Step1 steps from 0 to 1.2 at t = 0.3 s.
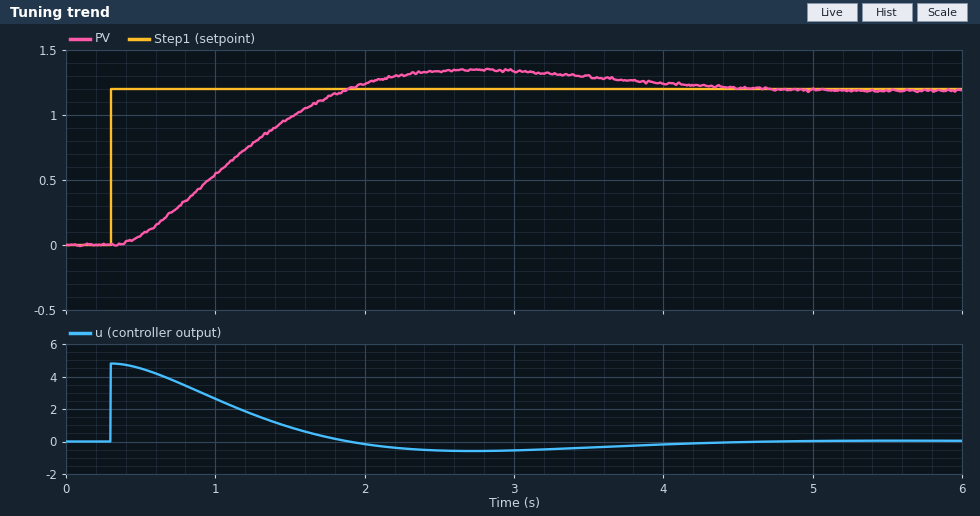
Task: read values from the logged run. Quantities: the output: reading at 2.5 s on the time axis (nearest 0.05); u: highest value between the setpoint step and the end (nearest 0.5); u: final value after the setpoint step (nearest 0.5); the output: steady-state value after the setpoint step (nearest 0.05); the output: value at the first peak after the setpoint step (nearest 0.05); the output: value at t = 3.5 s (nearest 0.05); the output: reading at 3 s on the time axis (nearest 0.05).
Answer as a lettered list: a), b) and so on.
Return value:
a) 1.35
b) 5.0
c) 0.0
d) 1.20
e) 1.35
f) 1.30
g) 1.35
